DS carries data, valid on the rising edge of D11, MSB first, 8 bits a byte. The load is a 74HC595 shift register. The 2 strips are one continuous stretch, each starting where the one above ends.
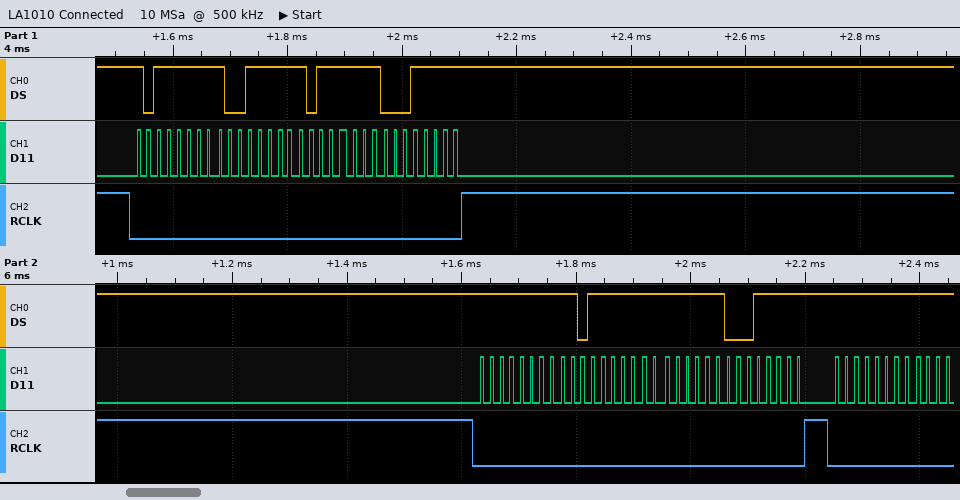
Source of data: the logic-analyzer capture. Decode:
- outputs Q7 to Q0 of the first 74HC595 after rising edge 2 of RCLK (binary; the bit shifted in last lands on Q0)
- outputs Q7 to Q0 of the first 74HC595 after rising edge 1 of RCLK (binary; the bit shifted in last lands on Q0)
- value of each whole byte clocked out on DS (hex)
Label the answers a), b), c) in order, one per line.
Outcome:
a) 00011111
b) 00011111
c) 0xBF 0x9F 0xBF 0x1F 0xFF 0xDF 0xFF 0x1F 0xFF
